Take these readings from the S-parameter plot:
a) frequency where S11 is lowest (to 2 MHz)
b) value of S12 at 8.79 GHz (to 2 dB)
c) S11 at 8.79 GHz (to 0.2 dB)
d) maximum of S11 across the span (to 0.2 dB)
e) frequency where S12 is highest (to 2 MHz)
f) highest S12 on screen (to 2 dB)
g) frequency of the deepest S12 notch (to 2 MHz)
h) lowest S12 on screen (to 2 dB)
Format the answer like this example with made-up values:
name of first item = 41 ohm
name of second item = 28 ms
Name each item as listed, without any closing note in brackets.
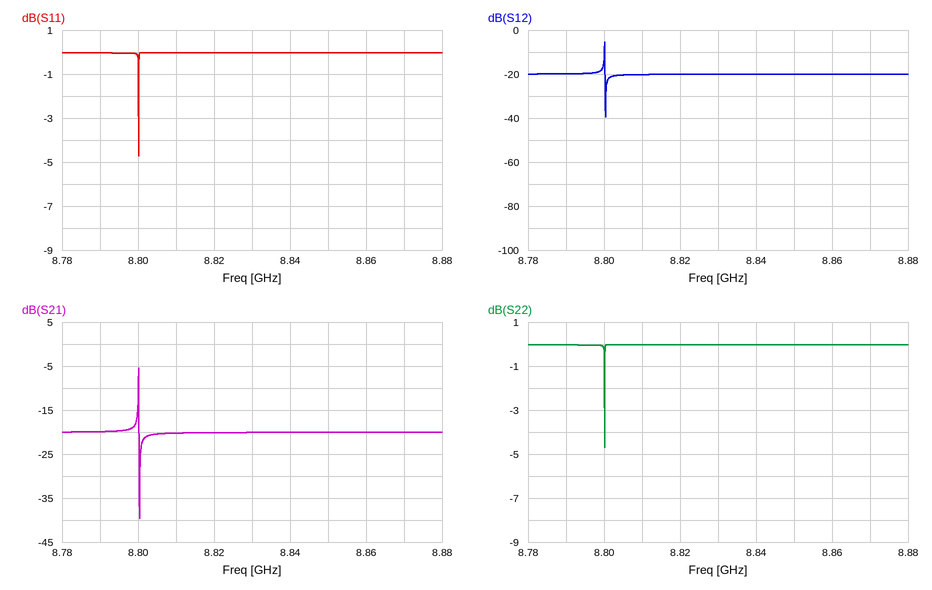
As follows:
frequency where S11 is lowest = 8.800 GHz
value of S12 at 8.79 GHz = -20 dB
S11 at 8.79 GHz = 0.0 dB
maximum of S11 across the span = 0.0 dB
frequency where S12 is highest = 8.800 GHz
highest S12 on screen = -6 dB
frequency of the deepest S12 notch = 8.800 GHz
lowest S12 on screen = -40 dB
